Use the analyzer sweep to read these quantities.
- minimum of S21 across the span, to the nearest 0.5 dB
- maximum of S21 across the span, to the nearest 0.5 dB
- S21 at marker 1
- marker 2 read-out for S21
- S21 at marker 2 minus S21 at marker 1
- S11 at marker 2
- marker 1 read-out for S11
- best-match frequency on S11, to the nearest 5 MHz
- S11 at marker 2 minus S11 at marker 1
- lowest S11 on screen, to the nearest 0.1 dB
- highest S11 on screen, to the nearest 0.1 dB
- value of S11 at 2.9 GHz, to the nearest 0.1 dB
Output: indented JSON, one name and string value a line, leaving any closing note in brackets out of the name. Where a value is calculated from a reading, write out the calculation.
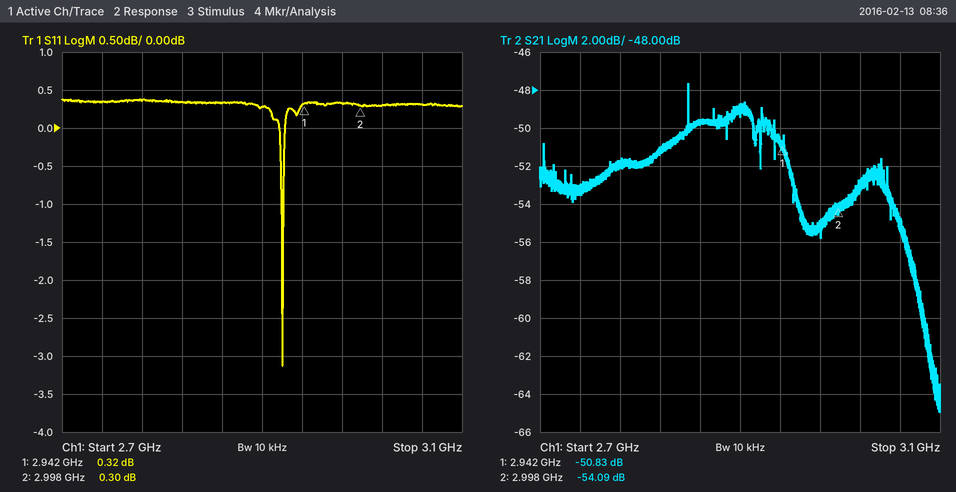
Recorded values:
{
  "minimum of S21 across the span, to the nearest 0.5 dB": "-65.0 dB",
  "maximum of S21 across the span, to the nearest 0.5 dB": "-47.5 dB",
  "S21 at marker 1": "-50.83 dB",
  "marker 2 read-out for S21": "-54.09 dB",
  "S21 at marker 2 minus S21 at marker 1": "-54.09 − (-50.83) = -3.26 dB",
  "S11 at marker 2": "0.30 dB",
  "marker 1 read-out for S11": "0.32 dB",
  "best-match frequency on S11, to the nearest 5 MHz": "2.920 GHz",
  "S11 at marker 2 minus S11 at marker 1": "0.3 − (0.32) = -0.02 dB",
  "lowest S11 on screen, to the nearest 0.1 dB": "-3.1 dB",
  "highest S11 on screen, to the nearest 0.1 dB": "0.4 dB",
  "value of S11 at 2.9 GHz, to the nearest 0.1 dB": "0.3 dB"
}
